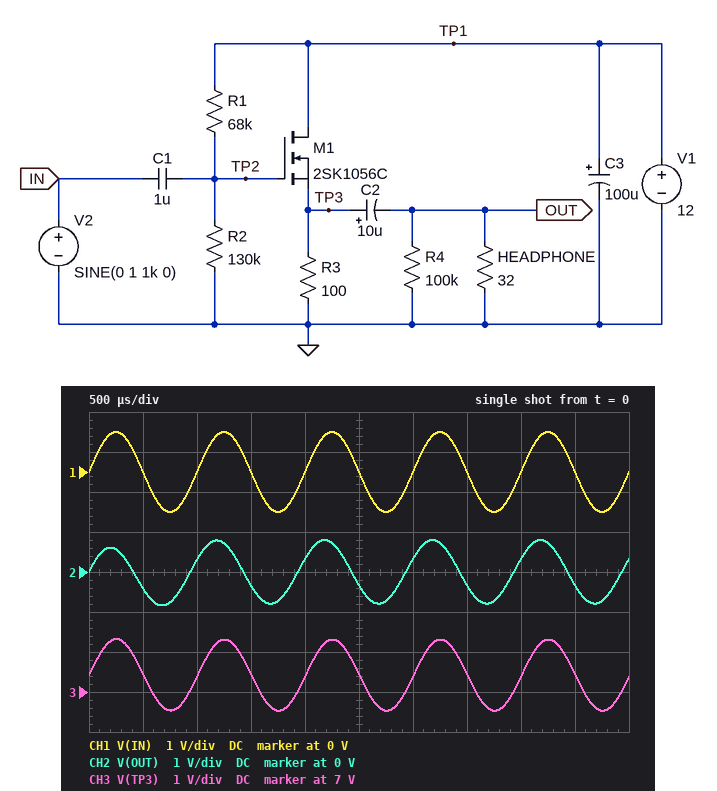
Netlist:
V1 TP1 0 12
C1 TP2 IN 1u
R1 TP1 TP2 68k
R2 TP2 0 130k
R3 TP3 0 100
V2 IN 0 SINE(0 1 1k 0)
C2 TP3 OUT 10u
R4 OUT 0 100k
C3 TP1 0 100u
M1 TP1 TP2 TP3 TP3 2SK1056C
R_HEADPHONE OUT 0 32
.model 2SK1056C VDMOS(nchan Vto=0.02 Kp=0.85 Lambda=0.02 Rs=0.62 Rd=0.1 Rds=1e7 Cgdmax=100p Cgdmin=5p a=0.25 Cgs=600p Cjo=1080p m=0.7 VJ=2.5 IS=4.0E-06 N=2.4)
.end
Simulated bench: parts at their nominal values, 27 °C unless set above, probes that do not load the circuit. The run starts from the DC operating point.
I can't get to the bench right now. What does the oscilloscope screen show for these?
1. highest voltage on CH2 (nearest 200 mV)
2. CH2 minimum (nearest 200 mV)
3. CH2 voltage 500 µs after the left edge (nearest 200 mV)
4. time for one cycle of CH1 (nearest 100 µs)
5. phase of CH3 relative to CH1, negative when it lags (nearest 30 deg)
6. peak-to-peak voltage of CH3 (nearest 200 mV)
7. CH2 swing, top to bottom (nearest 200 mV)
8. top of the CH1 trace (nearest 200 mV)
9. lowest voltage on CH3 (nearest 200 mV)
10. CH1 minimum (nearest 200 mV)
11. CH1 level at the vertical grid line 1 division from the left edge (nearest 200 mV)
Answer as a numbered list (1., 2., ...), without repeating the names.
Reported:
1. 800 mV
2. -800 mV
3. -400 mV
4. 1.0 ms
5. 0 deg
6. 1.8 V
7. 1.6 V
8. 1.0 V
9. 6.6 V
10. -1.0 V
11. 0 V
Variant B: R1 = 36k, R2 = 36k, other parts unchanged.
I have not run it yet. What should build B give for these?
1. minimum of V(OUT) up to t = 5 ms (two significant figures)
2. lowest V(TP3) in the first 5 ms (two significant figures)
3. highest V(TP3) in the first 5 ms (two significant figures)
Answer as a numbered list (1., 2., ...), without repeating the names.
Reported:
1. -820 mV
2. 4.7 V
3. 6.5 V
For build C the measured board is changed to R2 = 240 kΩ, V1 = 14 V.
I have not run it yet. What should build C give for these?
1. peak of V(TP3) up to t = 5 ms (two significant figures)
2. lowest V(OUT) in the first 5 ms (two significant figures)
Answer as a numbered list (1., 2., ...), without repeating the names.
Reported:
1. 11 V
2. -850 mV
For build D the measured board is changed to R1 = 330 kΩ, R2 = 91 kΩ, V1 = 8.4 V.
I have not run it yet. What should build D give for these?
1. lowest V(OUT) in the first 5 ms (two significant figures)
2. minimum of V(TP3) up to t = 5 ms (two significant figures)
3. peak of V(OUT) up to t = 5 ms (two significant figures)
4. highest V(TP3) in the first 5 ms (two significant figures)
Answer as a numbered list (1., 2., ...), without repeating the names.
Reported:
1. -470 mV
2. 1.2 V
3. 650 mV
4. 2.5 V
